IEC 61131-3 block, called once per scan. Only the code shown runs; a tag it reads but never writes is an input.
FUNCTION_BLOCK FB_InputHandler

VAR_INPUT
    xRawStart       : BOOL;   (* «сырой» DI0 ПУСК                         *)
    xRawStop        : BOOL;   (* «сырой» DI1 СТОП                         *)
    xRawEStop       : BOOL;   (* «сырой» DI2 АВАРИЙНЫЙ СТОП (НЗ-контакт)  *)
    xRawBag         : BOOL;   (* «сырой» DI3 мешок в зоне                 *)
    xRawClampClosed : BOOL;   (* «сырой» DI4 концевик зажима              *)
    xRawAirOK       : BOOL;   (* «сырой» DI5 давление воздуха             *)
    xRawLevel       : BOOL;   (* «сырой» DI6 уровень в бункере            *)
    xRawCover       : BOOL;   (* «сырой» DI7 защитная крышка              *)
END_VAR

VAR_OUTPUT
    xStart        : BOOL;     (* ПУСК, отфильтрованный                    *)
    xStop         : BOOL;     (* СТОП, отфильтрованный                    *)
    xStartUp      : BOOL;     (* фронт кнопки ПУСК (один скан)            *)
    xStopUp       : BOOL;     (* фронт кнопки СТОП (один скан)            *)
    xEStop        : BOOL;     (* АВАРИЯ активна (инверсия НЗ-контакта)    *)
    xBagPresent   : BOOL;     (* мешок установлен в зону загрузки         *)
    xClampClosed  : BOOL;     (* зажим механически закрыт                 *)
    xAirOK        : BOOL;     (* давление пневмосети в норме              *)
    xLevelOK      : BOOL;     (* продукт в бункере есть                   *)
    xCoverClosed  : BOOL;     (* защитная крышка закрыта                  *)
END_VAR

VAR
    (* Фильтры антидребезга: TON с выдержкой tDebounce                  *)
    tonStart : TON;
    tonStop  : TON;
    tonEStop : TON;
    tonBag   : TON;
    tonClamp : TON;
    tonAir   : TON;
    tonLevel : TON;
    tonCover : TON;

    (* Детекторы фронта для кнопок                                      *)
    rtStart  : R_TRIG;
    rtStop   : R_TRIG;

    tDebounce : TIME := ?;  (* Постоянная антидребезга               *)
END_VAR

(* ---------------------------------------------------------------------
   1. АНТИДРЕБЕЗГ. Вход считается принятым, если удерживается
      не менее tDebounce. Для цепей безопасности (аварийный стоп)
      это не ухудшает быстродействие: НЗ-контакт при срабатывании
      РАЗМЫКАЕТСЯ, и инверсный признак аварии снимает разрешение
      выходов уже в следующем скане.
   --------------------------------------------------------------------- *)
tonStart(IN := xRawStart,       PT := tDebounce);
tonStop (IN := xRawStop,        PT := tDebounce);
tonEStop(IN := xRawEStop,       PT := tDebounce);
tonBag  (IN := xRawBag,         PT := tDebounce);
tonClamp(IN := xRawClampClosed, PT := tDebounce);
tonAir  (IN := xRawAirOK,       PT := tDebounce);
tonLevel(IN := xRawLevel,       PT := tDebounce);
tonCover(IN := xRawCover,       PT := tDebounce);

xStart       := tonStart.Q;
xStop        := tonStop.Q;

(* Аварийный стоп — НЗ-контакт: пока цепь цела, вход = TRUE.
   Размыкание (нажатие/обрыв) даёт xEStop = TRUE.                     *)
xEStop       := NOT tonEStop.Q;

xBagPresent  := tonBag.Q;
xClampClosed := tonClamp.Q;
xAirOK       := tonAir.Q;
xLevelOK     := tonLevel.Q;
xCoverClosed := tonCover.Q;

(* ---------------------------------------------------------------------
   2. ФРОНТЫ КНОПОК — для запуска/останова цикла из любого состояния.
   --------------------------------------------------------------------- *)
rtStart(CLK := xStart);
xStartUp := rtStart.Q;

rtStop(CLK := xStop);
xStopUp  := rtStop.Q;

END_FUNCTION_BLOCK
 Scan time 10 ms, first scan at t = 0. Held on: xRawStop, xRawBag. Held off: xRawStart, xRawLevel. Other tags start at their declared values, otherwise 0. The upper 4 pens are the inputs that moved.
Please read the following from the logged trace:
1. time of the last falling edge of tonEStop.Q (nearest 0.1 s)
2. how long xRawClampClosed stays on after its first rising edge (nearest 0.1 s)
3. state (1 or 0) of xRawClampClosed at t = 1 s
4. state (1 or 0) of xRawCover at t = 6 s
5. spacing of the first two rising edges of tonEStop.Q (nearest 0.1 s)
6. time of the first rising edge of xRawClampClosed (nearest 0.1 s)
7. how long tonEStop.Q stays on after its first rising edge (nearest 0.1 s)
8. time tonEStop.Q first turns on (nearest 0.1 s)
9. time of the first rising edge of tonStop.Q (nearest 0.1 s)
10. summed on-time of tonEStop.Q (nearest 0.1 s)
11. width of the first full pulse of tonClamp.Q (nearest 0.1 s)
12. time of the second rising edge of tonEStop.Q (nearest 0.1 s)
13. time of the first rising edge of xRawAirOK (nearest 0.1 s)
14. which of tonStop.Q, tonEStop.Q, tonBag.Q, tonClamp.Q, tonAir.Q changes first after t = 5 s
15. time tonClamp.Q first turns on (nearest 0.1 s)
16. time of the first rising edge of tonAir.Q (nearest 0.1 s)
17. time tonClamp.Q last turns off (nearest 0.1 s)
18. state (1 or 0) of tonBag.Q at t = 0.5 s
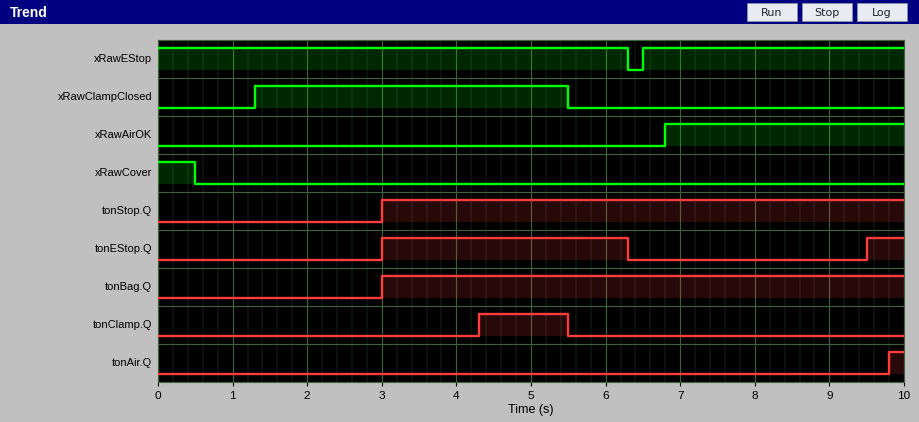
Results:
6.3 s
4.2 s
0
0
6.5 s
1.3 s
3.3 s
3.0 s
3.0 s
3.8 s
1.2 s
9.5 s
6.8 s
tonClamp.Q
4.3 s
9.8 s
5.5 s
0
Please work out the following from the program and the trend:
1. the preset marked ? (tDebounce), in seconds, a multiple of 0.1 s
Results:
3.0 s
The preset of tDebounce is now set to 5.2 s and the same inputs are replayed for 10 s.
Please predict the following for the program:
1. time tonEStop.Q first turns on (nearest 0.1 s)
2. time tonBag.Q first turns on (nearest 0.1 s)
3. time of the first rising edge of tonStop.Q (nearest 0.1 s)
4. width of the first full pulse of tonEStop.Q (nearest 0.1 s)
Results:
5.2 s
5.2 s
5.2 s
1.1 s
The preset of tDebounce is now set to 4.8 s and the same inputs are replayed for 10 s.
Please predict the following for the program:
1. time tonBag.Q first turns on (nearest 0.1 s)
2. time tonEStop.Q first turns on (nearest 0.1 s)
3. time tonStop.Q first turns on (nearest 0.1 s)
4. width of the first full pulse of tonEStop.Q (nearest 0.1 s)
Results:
4.8 s
4.8 s
4.8 s
1.5 s
